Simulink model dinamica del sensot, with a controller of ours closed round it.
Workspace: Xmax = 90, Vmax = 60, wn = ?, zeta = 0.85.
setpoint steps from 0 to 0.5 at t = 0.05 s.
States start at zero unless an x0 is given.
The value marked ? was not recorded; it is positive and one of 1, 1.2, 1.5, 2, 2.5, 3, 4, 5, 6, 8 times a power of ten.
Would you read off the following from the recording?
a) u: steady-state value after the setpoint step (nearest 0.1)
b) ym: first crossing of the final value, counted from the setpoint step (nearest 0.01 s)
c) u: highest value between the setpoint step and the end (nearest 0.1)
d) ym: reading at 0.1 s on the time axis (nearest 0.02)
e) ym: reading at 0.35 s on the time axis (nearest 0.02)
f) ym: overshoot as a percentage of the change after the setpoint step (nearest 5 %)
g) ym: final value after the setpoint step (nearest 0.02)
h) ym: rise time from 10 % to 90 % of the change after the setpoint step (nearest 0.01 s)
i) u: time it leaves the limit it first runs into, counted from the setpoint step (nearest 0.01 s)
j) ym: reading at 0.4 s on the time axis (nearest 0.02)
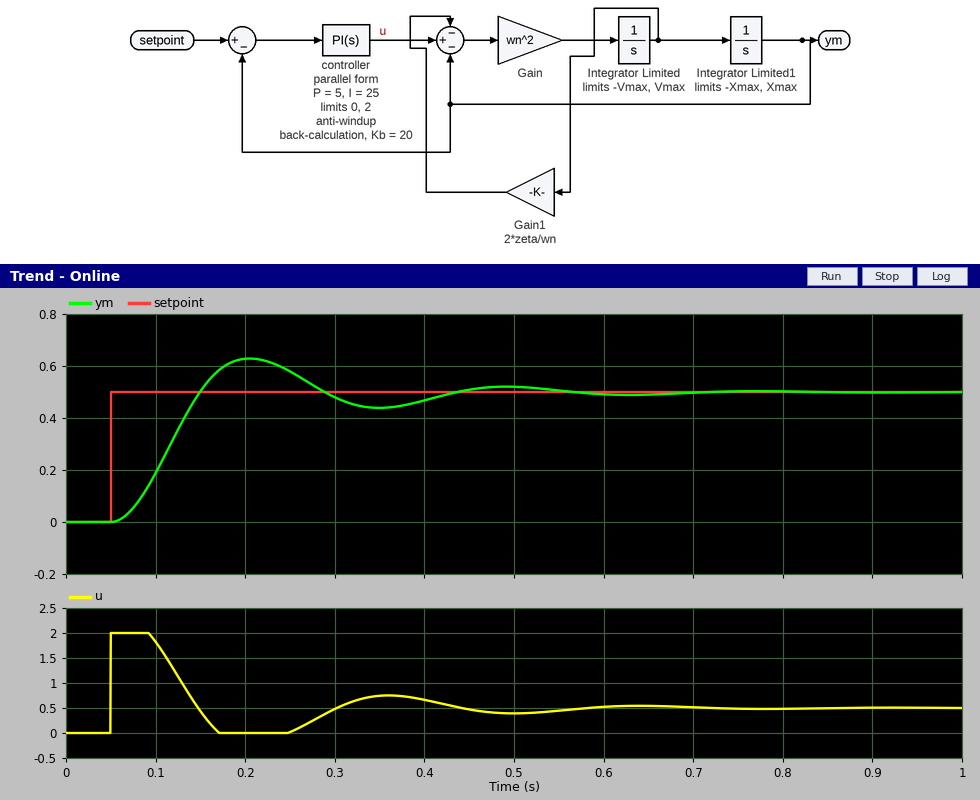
0.5
0.10 s
2.0
0.18
0.44
25 %
0.50
0.07 s
0.04 s
0.46
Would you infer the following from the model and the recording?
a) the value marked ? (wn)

10
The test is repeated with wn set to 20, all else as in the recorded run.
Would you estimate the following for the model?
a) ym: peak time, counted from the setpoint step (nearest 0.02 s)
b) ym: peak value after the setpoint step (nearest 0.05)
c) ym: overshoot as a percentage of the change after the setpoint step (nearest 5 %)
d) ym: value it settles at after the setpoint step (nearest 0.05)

0.08 s
0.60
20 %
0.50
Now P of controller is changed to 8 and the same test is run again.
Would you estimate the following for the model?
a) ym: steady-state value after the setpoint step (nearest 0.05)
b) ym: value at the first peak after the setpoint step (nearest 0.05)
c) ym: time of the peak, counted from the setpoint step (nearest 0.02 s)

0.50
0.55
0.14 s
